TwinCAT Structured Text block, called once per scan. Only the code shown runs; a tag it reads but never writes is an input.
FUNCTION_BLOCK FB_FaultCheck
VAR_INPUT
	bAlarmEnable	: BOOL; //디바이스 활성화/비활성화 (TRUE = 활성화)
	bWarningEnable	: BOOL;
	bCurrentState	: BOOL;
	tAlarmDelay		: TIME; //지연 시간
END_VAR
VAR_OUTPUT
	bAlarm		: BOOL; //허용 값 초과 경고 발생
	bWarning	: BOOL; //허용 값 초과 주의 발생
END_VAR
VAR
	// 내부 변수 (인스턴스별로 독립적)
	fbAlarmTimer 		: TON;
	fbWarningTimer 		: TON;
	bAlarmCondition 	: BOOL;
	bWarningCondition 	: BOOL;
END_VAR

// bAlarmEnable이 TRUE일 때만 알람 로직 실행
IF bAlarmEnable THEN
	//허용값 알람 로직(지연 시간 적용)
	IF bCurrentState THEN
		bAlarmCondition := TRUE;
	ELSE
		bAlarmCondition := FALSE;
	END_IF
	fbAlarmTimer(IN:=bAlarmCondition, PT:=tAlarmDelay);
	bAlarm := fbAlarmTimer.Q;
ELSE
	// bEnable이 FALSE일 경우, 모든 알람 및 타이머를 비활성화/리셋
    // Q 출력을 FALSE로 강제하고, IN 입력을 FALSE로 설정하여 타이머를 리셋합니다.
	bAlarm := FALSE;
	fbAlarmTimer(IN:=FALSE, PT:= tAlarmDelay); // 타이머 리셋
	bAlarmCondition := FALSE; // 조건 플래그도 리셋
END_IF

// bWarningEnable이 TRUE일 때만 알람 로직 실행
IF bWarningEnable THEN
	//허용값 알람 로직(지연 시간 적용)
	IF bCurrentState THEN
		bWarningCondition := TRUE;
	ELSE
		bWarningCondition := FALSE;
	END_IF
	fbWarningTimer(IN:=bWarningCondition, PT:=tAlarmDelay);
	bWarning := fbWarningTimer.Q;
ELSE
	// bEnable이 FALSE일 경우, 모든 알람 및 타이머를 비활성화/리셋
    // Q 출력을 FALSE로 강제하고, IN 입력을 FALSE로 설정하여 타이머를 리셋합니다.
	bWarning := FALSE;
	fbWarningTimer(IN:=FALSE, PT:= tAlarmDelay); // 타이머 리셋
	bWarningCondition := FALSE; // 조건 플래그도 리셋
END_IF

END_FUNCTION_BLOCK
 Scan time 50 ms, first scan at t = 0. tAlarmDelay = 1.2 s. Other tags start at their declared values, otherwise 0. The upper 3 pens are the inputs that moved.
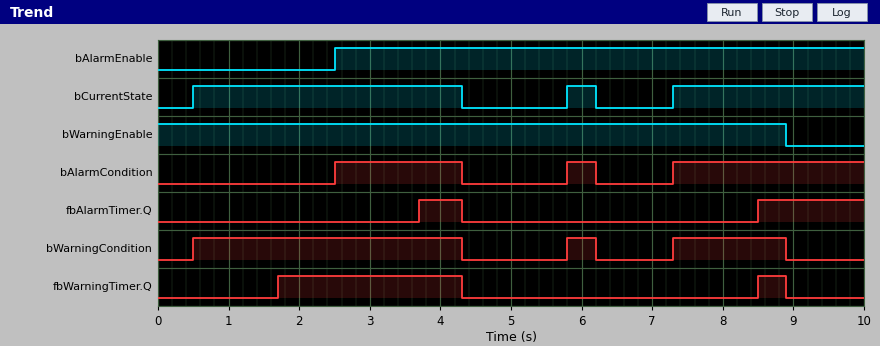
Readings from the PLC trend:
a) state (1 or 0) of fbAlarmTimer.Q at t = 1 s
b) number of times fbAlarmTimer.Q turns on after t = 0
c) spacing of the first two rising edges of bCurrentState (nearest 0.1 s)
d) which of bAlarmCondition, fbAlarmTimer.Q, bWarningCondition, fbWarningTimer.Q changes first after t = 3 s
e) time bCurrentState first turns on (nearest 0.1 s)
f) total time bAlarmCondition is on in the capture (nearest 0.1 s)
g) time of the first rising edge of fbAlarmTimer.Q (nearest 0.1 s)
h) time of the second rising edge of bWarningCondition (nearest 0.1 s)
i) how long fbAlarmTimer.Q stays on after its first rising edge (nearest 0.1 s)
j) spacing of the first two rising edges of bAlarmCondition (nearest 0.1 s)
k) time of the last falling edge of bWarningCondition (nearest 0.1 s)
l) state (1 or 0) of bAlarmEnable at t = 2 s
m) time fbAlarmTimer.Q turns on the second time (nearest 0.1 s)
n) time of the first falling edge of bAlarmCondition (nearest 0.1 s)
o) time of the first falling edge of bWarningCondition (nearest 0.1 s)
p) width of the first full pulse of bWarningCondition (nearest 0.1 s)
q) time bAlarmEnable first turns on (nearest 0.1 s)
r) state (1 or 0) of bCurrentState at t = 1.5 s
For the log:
0
2
5.3 s
fbAlarmTimer.Q
0.5 s
4.9 s
3.7 s
5.8 s
0.6 s
3.3 s
8.9 s
0
8.5 s
4.3 s
4.3 s
3.8 s
2.5 s
1
